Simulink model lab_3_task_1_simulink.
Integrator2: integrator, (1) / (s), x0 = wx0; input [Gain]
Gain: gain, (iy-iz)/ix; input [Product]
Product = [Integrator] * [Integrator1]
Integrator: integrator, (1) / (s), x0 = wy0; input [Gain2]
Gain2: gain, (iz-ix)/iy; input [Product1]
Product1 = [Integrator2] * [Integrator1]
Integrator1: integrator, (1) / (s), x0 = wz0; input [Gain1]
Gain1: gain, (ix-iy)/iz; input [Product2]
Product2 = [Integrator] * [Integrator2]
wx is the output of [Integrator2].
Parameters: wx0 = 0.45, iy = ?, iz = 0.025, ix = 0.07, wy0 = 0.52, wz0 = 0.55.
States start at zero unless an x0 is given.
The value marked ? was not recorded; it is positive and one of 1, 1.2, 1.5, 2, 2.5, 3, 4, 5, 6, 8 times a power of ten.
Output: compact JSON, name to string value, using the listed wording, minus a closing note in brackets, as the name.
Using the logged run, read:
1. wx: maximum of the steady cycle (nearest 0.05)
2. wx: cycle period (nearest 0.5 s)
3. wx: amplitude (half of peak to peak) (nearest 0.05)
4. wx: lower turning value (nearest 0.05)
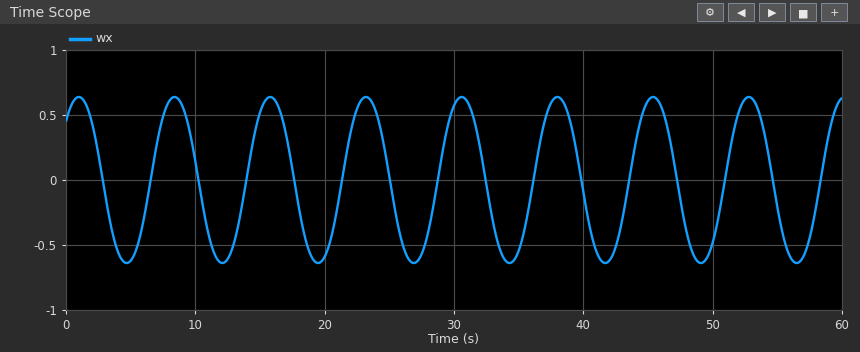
{"wx: maximum of the steady cycle": "0.65", "wx: cycle period": "7.5 s", "wx: amplitude (half of peak to peak)": "0.65", "wx: lower turning value": "-0.65"}
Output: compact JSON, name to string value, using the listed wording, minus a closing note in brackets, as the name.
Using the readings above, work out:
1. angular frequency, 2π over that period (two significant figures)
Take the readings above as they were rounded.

{"angular frequency, 2π over that period": "0.84 rad/s"}
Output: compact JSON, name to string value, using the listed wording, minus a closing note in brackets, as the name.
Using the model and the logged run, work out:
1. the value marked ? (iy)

{"the value marked ?": "0.12"}
